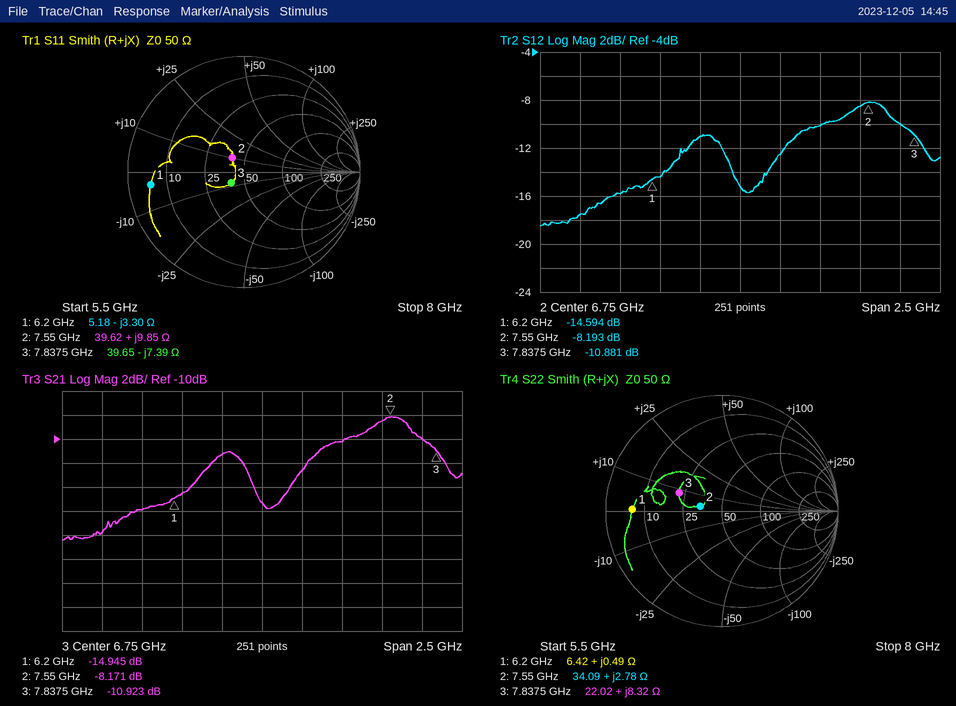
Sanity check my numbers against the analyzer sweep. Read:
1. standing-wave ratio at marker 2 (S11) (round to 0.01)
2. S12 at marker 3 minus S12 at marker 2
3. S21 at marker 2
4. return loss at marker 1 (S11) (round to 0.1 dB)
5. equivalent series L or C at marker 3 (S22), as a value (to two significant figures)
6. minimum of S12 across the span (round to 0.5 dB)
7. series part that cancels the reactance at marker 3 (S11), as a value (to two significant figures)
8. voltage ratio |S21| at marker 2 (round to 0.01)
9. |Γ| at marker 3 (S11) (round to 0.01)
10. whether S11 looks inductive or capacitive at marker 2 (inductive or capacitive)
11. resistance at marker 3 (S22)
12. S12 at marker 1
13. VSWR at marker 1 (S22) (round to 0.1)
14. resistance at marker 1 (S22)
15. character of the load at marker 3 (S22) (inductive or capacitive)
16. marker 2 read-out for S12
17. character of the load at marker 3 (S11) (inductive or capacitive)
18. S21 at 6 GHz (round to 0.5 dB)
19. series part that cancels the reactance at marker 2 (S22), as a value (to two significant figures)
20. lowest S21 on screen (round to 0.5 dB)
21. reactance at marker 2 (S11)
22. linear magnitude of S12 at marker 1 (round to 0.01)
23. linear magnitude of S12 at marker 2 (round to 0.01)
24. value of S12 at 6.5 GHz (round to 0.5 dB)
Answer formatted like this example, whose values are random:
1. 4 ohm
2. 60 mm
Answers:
1. 1.38
2. -2.688 dB
3. -8.171 dB
4. 1.8 dB
5. 170 pH
6. -18.5 dB
7. 150 pH
8. 0.39
9. 0.14
10. inductive
11. 22.02 Ω
12. -14.594 dB
13. 7.8
14. 6.42 Ω
15. inductive
16. -8.193 dB
17. capacitive
18. -16.0 dB
19. 7.6 pF
20. -18.5 dB
21. +9.85 Ω
22. 0.19
23. 0.39
24. -11.0 dB
